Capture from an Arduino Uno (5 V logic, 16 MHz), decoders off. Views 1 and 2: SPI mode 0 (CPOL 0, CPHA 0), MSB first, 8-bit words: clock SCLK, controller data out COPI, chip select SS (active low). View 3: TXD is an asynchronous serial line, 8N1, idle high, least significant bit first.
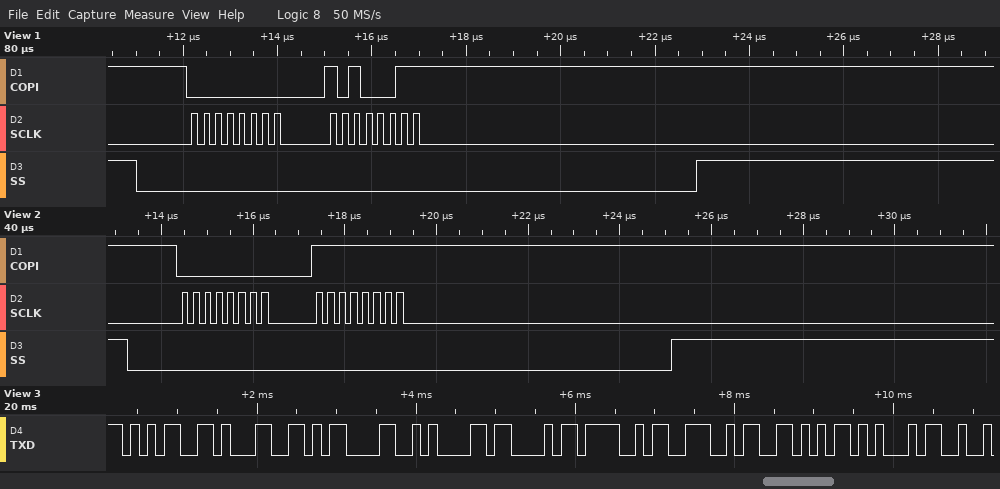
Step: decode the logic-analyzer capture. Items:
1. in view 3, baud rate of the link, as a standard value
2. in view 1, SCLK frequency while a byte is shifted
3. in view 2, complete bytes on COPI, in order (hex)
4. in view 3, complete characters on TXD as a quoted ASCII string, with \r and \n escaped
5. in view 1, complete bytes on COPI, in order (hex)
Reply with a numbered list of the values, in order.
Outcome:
1. 9600 baud
2. 4 MHz
3. 0x00 0xFF
4. "51\r\nCONVE"
5. 00 A3
